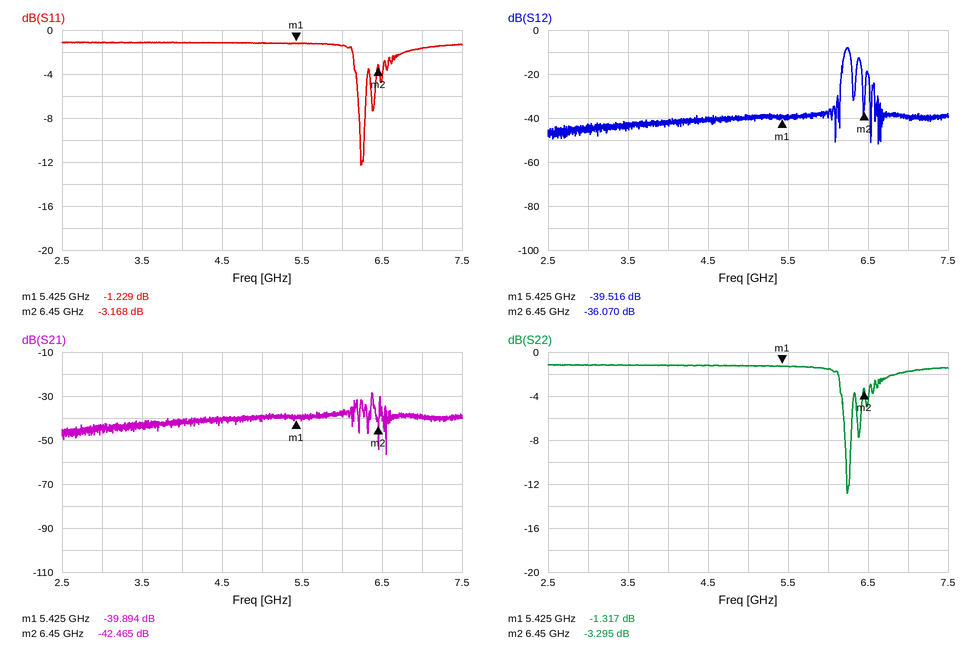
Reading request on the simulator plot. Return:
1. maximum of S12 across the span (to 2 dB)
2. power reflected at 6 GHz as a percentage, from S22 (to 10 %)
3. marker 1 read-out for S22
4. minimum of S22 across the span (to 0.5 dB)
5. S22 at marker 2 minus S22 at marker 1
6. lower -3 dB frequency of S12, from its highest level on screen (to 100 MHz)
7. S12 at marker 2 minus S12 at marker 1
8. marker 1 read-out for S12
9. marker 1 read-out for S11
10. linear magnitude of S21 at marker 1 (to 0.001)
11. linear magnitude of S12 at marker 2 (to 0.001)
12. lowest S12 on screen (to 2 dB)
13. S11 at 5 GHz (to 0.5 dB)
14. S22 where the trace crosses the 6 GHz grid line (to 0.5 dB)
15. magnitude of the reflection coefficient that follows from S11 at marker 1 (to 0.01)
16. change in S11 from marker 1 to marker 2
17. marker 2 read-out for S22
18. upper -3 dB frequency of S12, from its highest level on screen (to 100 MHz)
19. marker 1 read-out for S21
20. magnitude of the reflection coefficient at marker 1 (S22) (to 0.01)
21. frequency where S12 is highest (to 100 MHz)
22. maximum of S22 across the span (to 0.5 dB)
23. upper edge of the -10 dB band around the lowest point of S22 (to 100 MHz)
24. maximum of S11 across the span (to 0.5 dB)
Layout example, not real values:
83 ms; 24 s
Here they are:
-8 dB; 70 %; -1.317 dB; -13.0 dB; -1.978 dB; 6.2 GHz; 3.446 dB; -39.516 dB; -1.229 dB; 0.010; 0.016; -52 dB; -1.0 dB; -1.5 dB; 0.87; -1.939 dB; -3.295 dB; 6.3 GHz; -39.894 dB; 0.86; 6.2 GHz; -1.0 dB; 6.3 GHz; -1.0 dB
